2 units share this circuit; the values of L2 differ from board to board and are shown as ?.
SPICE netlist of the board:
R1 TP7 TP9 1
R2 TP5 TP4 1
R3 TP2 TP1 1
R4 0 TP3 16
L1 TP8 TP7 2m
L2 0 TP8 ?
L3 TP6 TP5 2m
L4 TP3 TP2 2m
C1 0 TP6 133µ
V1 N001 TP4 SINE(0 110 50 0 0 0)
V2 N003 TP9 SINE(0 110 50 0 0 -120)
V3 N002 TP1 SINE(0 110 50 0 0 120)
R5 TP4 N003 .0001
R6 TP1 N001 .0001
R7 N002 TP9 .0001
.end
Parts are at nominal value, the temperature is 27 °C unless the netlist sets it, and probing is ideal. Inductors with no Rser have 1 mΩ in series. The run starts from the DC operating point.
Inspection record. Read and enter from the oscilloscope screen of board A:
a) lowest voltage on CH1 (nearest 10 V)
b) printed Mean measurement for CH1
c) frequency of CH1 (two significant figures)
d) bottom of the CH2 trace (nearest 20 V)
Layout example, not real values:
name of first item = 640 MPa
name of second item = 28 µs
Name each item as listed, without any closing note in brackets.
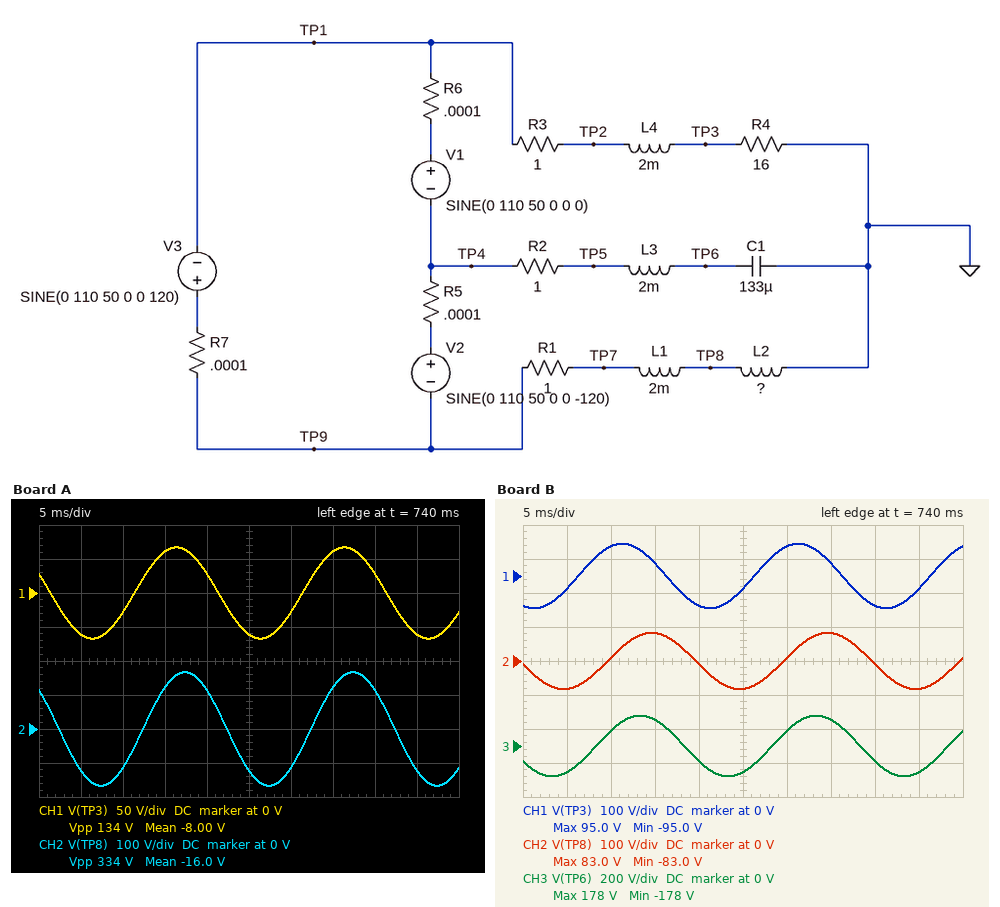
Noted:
lowest voltage on CH1 = -70 V
printed Mean measurement for CH1 = -8.00 V
frequency of CH1 = 50 Hz
bottom of the CH2 trace = -160 V
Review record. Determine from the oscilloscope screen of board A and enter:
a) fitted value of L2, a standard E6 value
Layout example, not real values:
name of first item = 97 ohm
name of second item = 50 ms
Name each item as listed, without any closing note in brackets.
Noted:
fitted value of L2, a standard E6 value = 68 mH
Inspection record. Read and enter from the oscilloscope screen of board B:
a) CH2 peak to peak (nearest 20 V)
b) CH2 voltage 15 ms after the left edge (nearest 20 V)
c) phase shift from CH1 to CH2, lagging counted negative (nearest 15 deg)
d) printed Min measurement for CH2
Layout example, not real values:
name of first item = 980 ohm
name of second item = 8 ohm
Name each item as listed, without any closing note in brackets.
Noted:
CH2 peak to peak = 160 V
CH2 voltage 15 ms after the left edge = 80 V
phase shift from CH1 to CH2, lagging counted negative = -60 deg
printed Min measurement for CH2 = -83.0 V
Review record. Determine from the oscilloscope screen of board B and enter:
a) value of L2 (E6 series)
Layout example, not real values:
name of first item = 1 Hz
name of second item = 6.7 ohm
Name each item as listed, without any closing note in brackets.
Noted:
value of L2 = 22 mH
